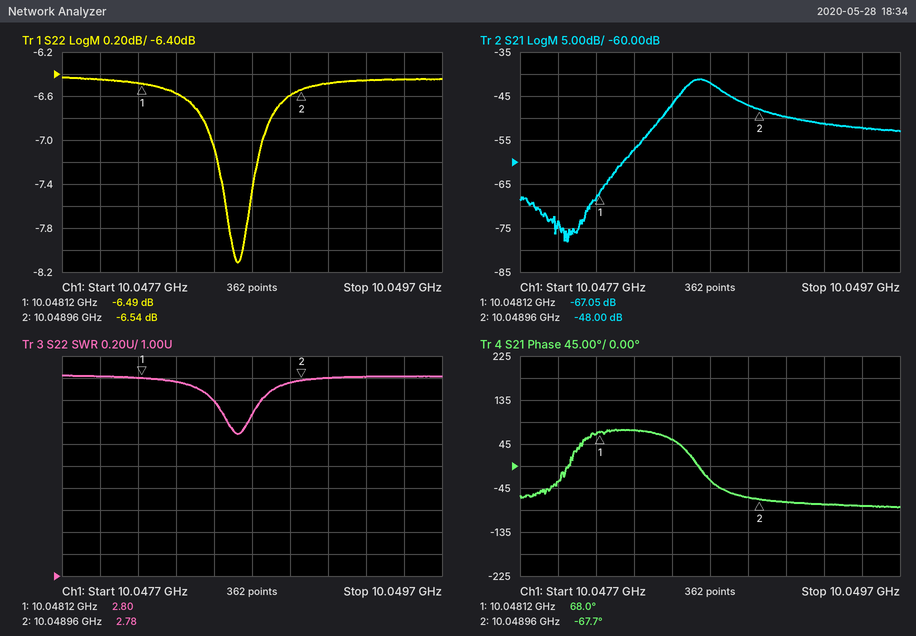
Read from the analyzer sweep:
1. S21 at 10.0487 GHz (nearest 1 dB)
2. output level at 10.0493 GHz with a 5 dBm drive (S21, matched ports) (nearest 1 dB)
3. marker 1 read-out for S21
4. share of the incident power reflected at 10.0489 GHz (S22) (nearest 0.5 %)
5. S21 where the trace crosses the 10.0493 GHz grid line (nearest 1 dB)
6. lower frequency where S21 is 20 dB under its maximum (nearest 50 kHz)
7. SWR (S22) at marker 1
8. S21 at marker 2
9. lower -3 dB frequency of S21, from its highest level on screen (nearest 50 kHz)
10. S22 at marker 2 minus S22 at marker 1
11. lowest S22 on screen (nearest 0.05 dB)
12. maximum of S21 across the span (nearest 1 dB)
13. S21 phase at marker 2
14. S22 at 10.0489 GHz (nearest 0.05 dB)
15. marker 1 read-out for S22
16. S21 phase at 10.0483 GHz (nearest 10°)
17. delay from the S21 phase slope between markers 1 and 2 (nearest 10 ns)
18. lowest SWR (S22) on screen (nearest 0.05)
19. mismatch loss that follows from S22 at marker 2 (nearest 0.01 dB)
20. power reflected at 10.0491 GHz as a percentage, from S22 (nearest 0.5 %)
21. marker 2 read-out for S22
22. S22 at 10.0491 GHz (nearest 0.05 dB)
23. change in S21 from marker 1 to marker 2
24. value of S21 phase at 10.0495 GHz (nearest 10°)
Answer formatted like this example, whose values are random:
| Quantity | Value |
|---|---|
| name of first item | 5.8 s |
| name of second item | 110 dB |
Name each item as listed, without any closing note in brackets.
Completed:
| Quantity | Value |
|---|---|
| S21 at 10.0487 GHz | -42 dB |
| output level at 10.0493 GHz with a 5 dBm drive (S21, matched ports) | -46 dBm |
| marker 1 read-out for S21 | -67.05 dB |
| share of the incident power reflected at 10.0489 GHz (S22) | 22.0 % |
| S21 where the trace crosses the 10.0493 GHz grid line | -51 dB |
| lower frequency where S21 is 20 dB under its maximum | 10.04820 GHz |
| SWR (S22) at marker 1 | 2.80 |
| S21 at marker 2 | -48.00 dB |
| lower -3 dB frequency of S21, from its highest level on screen | 10.04855 GHz |
| S22 at marker 2 minus S22 at marker 1 | -0.05 dB |
| lowest S22 on screen | -8.10 dB |
| maximum of S21 across the span | -41 dB |
| S21 phase at marker 2 | -67.7° |
| S22 at 10.0489 GHz | -6.60 dB |
| marker 1 read-out for S22 | -6.49 dB |
| S21 phase at 10.0483 GHz | 70° |
| delay from the S21 phase slope between markers 1 and 2 | 450 ns |
| lowest SWR (S22) on screen | 2.30 |
| mismatch loss that follows from S22 at marker 2 | 1.09 dB |
| power reflected at 10.0491 GHz as a percentage, from S22 | 22.5 % |
| marker 2 read-out for S22 | -6.54 dB |
| S22 at 10.0491 GHz | -6.50 dB |
| change in S21 from marker 1 to marker 2 | 19.05 dB |
| value of S21 phase at 10.0495 GHz | -80° |
